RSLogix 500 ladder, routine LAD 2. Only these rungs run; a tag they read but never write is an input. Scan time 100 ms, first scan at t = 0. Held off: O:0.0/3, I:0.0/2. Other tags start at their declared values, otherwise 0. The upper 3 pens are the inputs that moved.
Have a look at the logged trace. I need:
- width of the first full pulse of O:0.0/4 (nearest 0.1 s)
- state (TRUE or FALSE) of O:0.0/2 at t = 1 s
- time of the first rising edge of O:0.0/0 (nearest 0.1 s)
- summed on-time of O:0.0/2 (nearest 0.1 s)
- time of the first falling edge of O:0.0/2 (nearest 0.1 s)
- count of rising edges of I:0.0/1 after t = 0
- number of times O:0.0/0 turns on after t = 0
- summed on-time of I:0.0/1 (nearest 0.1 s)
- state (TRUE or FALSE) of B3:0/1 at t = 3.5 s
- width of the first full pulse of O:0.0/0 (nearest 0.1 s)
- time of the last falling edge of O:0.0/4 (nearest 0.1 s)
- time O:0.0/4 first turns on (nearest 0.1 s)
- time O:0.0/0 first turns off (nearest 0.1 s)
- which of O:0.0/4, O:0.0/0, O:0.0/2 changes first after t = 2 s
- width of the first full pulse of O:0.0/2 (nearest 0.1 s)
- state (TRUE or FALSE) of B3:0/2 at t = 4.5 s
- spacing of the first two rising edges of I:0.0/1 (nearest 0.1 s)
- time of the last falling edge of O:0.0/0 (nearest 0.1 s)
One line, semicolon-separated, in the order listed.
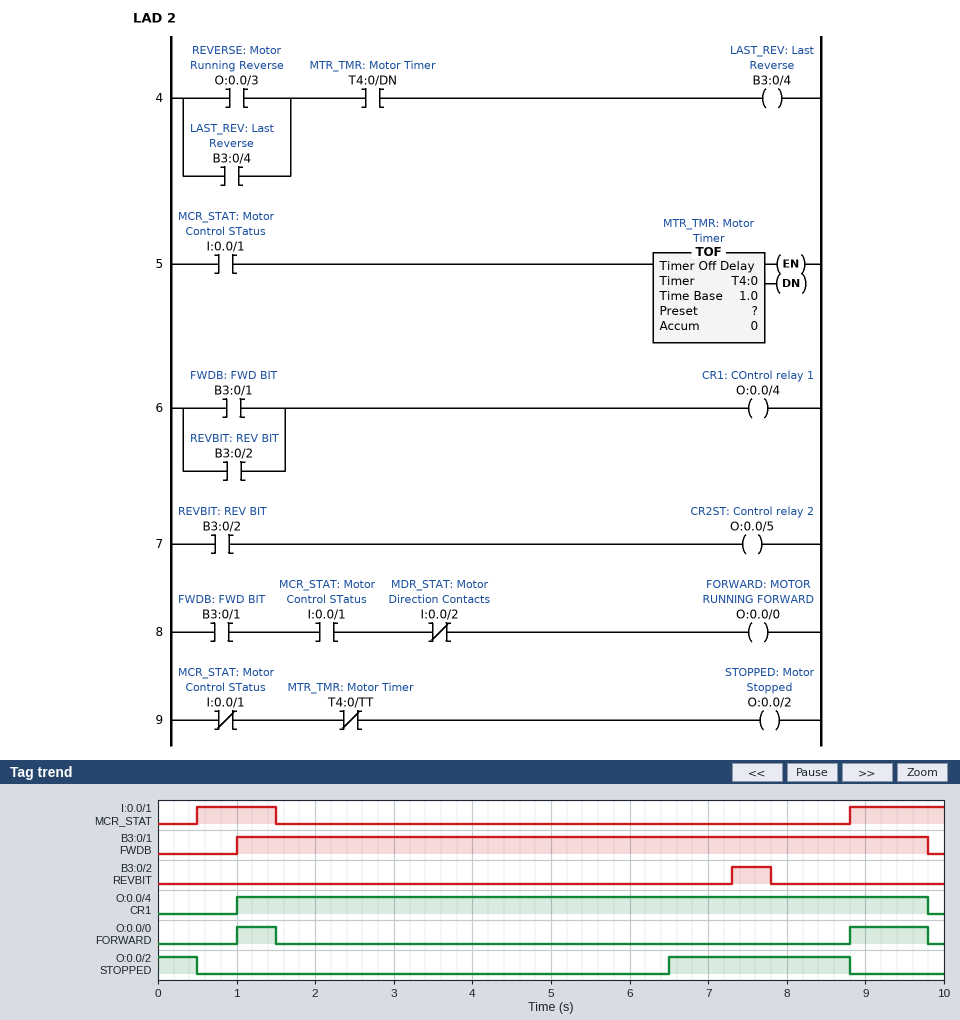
8.8 s; FALSE; 1.0 s; 2.8 s; 0.5 s; 2; 2; 2.2 s; TRUE; 0.5 s; 9.8 s; 1.0 s; 1.5 s; O:0.0/2; 2.3 s; FALSE; 8.3 s; 9.8 s
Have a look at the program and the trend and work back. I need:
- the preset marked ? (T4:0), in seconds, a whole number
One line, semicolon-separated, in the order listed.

5 s
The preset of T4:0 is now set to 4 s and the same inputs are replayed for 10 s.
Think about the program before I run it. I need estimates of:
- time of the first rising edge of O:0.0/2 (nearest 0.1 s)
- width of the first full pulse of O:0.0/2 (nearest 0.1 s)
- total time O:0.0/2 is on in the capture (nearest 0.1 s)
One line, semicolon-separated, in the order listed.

5.5 s; 3.3 s; 3.8 s
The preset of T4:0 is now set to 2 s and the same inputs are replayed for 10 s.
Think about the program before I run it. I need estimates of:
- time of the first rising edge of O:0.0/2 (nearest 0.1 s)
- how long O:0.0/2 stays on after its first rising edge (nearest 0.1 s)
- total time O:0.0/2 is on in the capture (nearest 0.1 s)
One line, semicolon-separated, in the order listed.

3.5 s; 5.3 s; 5.8 s
